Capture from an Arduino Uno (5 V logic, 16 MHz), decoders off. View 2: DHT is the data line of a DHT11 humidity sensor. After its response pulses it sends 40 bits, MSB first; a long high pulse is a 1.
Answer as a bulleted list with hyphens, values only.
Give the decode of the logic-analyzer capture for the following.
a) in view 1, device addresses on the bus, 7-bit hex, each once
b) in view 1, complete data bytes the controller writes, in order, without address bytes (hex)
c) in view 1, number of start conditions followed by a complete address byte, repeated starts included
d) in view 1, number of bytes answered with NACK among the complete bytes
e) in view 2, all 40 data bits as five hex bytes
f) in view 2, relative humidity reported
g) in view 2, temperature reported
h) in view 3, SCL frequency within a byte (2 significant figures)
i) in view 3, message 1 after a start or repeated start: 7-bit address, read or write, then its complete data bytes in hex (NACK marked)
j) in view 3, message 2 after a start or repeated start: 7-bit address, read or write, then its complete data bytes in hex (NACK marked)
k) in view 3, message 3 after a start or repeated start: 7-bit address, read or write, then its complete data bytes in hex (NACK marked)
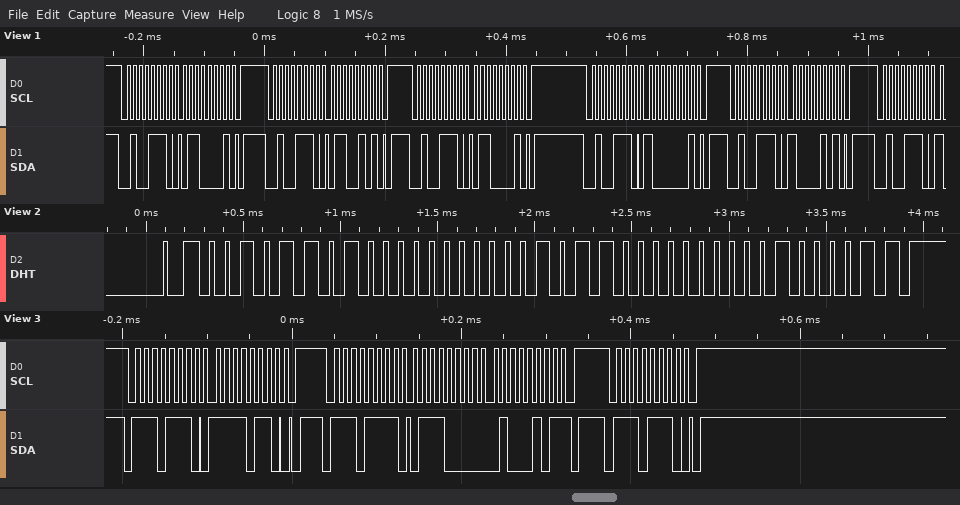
- 0x27
- 61 65 61 81 85
- 6
- 0
- 2D 00 16 00 43
- 45 %
- 22.0 °C
- 100 kHz
- 0x77 write: F6
- 0x77 read: 70 45 NACK
- 0x77 write
